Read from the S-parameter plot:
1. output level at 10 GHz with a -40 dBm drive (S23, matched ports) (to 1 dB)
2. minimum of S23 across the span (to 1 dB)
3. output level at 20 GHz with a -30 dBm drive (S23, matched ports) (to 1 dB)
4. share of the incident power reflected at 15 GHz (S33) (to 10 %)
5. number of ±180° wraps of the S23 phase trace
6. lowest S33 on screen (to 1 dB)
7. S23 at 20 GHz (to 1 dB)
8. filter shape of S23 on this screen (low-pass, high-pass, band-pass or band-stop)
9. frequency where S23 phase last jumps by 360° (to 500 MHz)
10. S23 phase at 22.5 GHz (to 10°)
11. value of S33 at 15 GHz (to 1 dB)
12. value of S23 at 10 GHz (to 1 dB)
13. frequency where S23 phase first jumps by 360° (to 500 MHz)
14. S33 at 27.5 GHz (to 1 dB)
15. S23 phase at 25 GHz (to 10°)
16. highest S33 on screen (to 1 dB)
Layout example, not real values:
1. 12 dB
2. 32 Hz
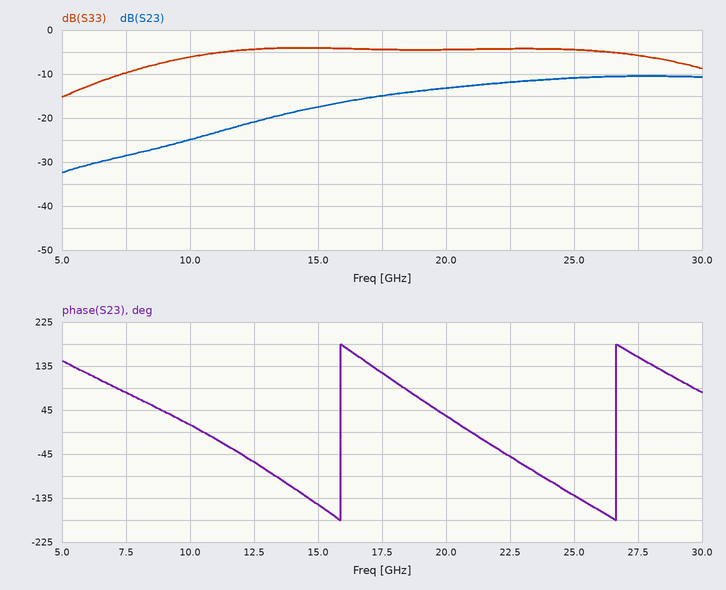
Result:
1. -65 dBm
2. -32 dB
3. -43 dBm
4. 40 %
5. 2
6. -15 dB
7. -13 dB
8. high-pass
9. 26.5 GHz
10. -50°
11. -4 dB
12. -25 dB
13. 16.0 GHz
14. -6 dB
15. -130°
16. -4 dB
